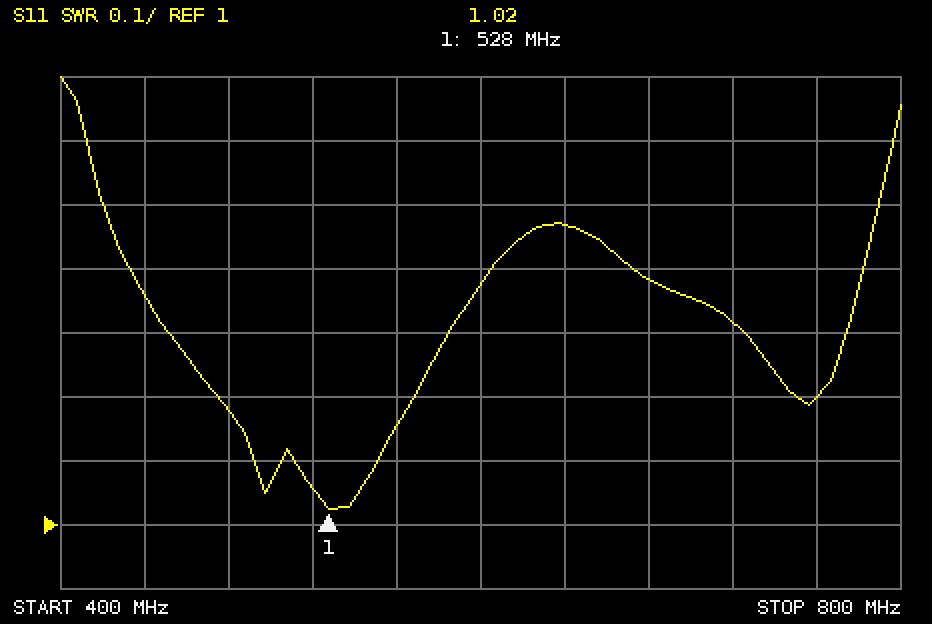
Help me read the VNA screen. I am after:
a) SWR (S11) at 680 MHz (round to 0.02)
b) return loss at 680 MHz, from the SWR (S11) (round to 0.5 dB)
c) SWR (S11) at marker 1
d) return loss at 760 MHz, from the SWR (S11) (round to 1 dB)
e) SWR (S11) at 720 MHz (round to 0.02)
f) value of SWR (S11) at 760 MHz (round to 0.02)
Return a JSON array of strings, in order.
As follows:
["1.38", "16.0 dB", "1.02", "21 dB", "1.32", "1.20"]
